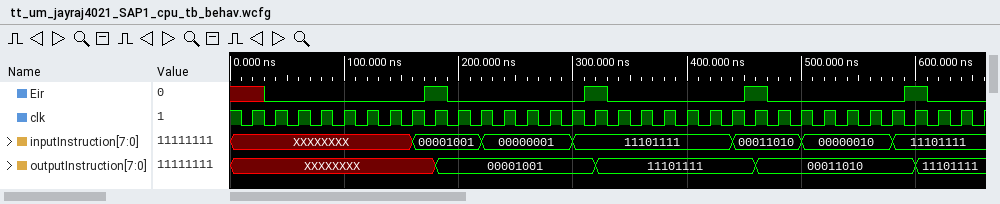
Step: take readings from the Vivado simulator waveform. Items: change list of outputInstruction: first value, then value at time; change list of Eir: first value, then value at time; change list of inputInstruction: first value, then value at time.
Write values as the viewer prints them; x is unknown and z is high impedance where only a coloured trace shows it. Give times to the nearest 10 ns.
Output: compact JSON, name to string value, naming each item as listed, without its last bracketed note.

{"change list of outputInstruction: first value, then value at time": "XXXXXXXX, 00001001 at 180 ns, 11101111 at 320 ns, 00011010 at 460 ns, 11101111 at 600 ns", "change list of Eir: first value, then value at time": "x, 0 at 30 ns, 1 at 170 ns, 0 at 190 ns, 1 at 310 ns, 0 at 330 ns, 1 at 450 ns, 0 at 470 ns, 1 at 590 ns, 0 at 610 ns", "change list of inputInstruction: first value, then value at time": "XXXXXXXX, 00001001 at 160 ns, 00000001 at 220 ns, 11101111 at 300 ns, 00011010 at 440 ns, 00000010 at 500 ns, 11101111 at 580 ns"}
